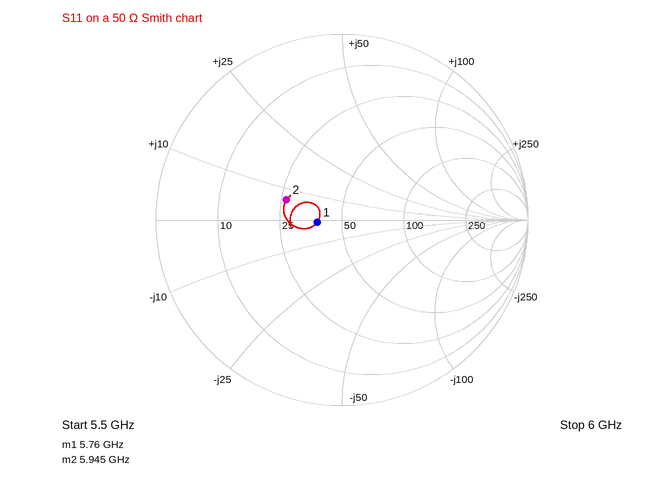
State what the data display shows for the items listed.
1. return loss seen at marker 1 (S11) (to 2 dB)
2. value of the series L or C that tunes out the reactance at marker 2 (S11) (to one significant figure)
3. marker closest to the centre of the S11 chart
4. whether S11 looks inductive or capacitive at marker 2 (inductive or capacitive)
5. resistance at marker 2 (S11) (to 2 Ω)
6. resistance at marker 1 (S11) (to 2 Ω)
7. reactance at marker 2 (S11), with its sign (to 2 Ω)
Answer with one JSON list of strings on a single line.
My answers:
["18 dB", "4 pF", "marker 1", "inductive", "26 Ω", "38 Ω", "+6 Ω"]
